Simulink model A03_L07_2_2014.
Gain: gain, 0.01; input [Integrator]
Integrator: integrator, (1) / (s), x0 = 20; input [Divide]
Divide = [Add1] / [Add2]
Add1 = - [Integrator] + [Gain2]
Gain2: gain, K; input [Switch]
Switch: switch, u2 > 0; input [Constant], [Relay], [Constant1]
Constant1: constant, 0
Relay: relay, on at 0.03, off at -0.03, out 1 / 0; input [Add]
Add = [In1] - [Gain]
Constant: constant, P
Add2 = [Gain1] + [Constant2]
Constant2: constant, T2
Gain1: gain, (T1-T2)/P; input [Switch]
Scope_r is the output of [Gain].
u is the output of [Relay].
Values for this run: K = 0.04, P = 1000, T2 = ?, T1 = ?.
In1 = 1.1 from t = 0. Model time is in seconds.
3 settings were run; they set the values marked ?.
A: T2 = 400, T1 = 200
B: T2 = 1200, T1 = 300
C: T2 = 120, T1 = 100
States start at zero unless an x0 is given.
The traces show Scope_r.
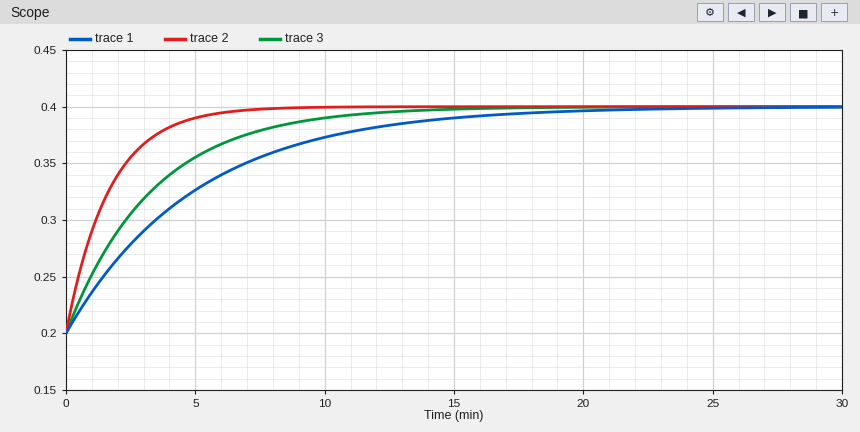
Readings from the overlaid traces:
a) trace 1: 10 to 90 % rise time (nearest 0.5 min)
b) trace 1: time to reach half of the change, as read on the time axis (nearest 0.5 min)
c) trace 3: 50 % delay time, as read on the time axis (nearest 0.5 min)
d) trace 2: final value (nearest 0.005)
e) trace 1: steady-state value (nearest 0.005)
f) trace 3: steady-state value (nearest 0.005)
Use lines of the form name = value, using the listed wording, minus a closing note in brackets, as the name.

trace 1: 10 to 90 % rise time = 11.0 min
trace 1: time to reach half of the change, as read on the time axis = 3.5 min
trace 3: 50 % delay time, as read on the time axis = 2.5 min
trace 2: final value = 0.400
trace 1: steady-state value = 0.400
trace 3: steady-state value = 0.400
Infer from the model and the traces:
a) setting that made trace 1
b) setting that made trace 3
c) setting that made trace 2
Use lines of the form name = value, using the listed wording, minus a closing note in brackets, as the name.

setting that made trace 1 = B
setting that made trace 3 = A
setting that made trace 2 = C
